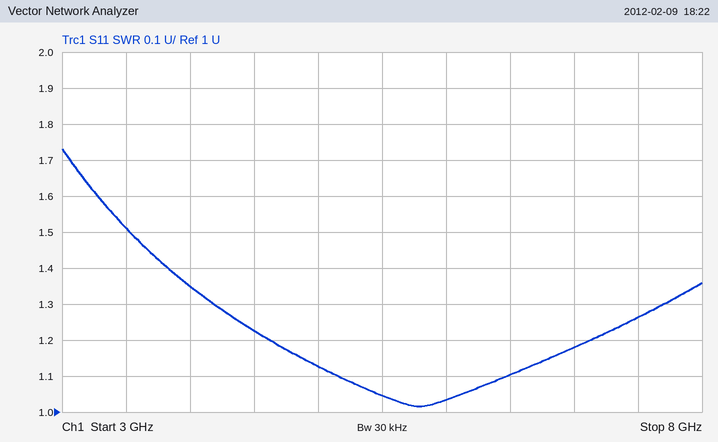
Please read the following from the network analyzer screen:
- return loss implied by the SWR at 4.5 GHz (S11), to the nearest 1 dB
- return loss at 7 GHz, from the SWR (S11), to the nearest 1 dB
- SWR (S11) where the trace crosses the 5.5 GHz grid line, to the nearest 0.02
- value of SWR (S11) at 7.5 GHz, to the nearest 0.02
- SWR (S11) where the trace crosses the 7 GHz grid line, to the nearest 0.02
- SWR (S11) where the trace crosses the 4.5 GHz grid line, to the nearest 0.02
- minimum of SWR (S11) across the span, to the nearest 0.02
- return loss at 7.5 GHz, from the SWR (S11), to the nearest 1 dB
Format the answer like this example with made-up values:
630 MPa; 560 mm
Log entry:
20 dB; 22 dB; 1.04; 1.26; 1.18; 1.22; 1.02; 19 dB
